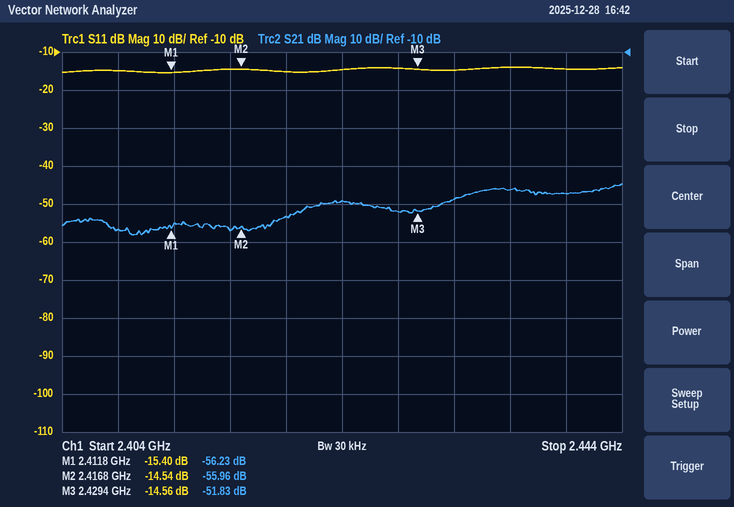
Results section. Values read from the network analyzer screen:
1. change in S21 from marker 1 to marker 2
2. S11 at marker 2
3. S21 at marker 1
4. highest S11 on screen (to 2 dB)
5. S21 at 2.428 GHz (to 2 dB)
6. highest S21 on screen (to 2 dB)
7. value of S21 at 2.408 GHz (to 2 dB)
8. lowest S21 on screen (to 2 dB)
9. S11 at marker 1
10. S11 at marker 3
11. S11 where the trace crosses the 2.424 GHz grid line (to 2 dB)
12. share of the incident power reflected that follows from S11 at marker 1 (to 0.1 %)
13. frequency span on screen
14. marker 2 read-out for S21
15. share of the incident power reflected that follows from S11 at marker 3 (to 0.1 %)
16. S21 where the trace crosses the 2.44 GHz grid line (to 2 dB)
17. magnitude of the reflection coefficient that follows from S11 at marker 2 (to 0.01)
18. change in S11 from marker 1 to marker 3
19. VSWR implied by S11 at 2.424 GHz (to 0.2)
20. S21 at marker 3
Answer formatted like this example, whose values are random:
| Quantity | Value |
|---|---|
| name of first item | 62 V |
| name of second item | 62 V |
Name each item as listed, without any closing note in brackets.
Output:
| Quantity | Value |
|---|---|
| change in S21 from marker 1 to marker 2 | 0.27 dB |
| S11 at marker 2 | -14.54 dB |
| S21 at marker 1 | -56.23 dB |
| highest S11 on screen | -14 dB |
| S21 at 2.428 GHz | -52 dB |
| highest S21 on screen | -44 dB |
| value of S21 at 2.408 GHz | -56 dB |
| lowest S21 on screen | -58 dB |
| S11 at marker 1 | -15.40 dB |
| S11 at marker 3 | -14.56 dB |
| S11 where the trace crosses the 2.424 GHz grid line | -14 dB |
| share of the incident power reflected that follows from S11 at marker 1 | 2.9 % |
| frequency span on screen | 40 MHz |
| marker 2 read-out for S21 | -55.96 dB |
| share of the incident power reflected that follows from S11 at marker 3 | 3.5 % |
| S21 where the trace crosses the 2.44 GHz grid line | -48 dB |
| magnitude of the reflection coefficient that follows from S11 at marker 2 | 0.19 |
| change in S11 from marker 1 to marker 3 | 0.84 dB |
| VSWR implied by S11 at 2.424 GHz | 1.4 |
| S21 at marker 3 | -51.83 dB |
